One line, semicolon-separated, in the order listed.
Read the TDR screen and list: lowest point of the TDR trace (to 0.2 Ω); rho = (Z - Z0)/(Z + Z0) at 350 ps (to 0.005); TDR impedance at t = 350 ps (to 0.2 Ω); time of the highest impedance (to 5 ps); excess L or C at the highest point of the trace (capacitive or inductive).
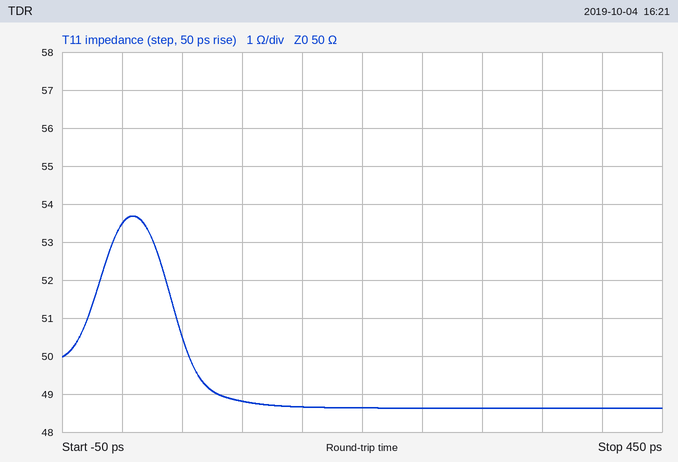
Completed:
48.6 Ω; -0.015; 48.6 Ω; 10 ps; inductive
